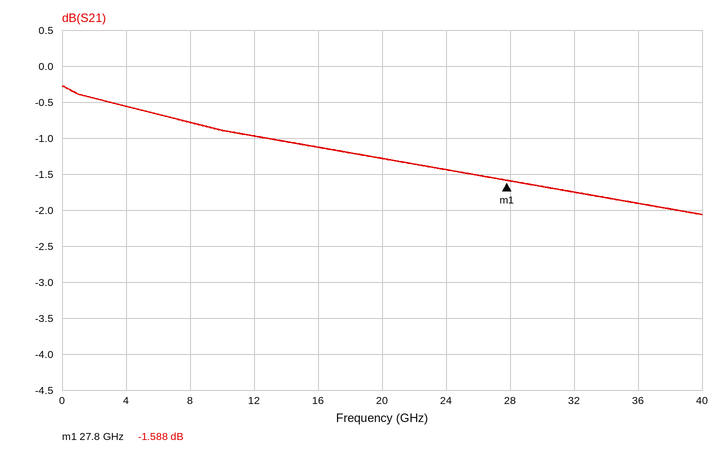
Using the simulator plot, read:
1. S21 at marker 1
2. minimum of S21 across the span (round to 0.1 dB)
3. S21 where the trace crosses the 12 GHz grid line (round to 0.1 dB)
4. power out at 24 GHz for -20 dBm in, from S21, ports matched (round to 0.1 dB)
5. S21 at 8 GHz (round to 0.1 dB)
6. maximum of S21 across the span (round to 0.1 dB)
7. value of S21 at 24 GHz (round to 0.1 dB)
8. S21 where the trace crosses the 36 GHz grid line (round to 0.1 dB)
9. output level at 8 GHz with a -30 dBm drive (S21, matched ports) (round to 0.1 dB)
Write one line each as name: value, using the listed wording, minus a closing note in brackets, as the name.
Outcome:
S21 at marker 1: -1.588 dB
minimum of S21 across the span: -2.1 dB
S21 where the trace crosses the 12 GHz grid line: -1.0 dB
power out at 24 GHz for -20 dBm in, from S21, ports matched: -21.4 dBm
S21 at 8 GHz: -0.8 dB
maximum of S21 across the span: -0.3 dB
value of S21 at 24 GHz: -1.4 dB
S21 where the trace crosses the 36 GHz grid line: -1.9 dB
output level at 8 GHz with a -30 dBm drive (S21, matched ports): -30.8 dBm
